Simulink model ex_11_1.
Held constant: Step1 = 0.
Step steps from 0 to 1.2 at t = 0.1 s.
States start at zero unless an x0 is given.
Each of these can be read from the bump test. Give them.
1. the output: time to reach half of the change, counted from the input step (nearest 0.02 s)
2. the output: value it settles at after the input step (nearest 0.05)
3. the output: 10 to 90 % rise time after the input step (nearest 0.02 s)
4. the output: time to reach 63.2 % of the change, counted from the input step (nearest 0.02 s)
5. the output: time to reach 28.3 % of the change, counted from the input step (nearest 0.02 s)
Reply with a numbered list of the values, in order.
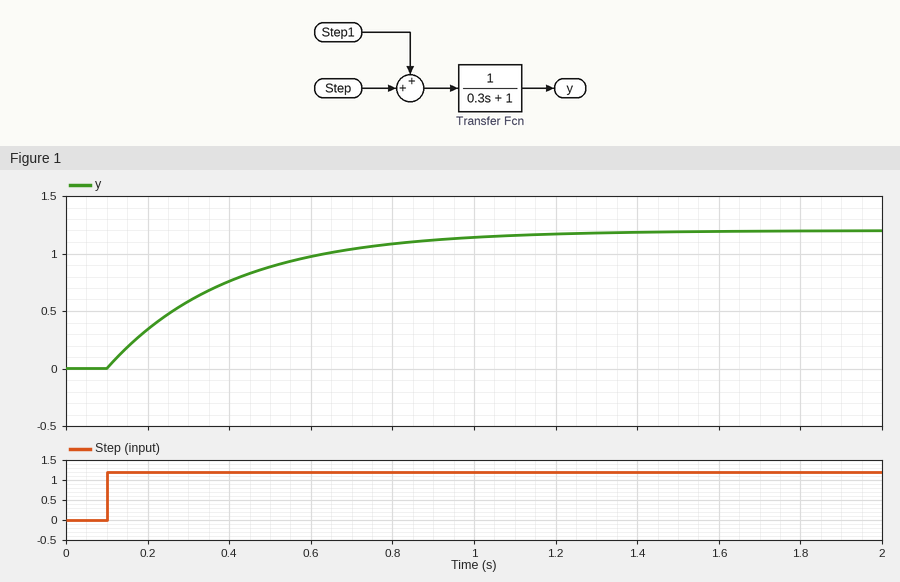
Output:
1. 0.20 s
2. 1.20
3. 0.66 s
4. 0.30 s
5. 0.10 s
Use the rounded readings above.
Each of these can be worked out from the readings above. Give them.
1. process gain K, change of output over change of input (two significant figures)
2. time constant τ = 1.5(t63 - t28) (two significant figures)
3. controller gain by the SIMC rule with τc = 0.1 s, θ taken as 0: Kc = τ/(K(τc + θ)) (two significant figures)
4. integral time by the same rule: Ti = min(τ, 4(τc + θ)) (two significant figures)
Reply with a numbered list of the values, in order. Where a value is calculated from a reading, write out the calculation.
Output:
1. (1.2 - 0) / 1.2 = 1.0
2. 1.5 × (0.3 - 0.1) = 0.30 s
3. 0.3 / (1 × (0.1 + 0)) = 3.0
4. min(0.3, 4 × (0.1 + 0)) = 0.30 s
